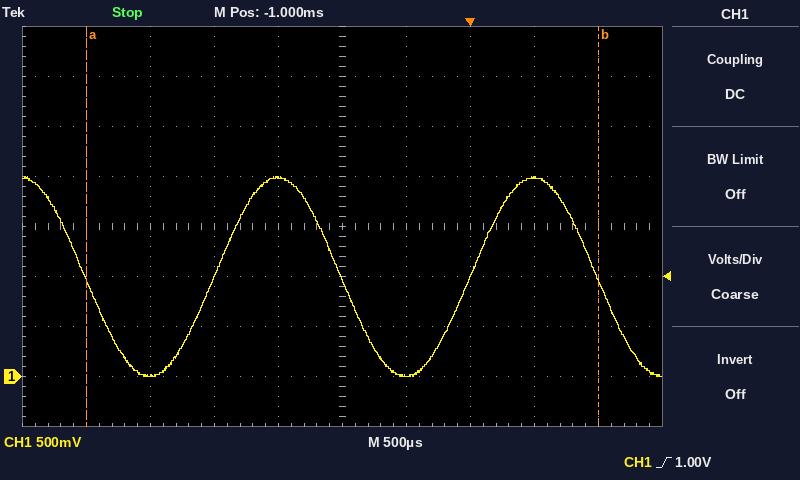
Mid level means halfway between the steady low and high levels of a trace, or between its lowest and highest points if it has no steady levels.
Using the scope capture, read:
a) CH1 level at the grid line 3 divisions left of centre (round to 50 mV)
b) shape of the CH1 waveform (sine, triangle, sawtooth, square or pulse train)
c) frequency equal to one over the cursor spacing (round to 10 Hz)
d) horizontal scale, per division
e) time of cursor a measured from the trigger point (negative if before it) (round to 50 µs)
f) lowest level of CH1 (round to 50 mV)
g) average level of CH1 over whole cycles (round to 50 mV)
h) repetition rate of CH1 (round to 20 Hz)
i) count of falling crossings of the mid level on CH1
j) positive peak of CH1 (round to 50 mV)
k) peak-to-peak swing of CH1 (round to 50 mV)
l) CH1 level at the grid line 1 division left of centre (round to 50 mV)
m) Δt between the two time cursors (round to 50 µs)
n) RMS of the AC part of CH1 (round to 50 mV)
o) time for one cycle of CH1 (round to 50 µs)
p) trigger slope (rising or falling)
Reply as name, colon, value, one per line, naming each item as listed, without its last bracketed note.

CH1 level at the grid line 3 divisions left of centre: 0 mV
shape of the CH1 waveform: sine
frequency equal to one over the cursor spacing: 250 Hz
horizontal scale, per division: 500 µs
time of cursor a measured from the trigger point (negative if before it): -3.00 ms
lowest level of CH1: 0 mV
average level of CH1 over whole cycles: 1.00 V
repetition rate of CH1: 500 Hz
count of falling crossings of the mid level on CH1: 3
positive peak of CH1: 2.00 V
peak-to-peak swing of CH1: 2.00 V
CH1 level at the grid line 1 division left of centre: 2.00 V
Δt between the two time cursors: 4.00 ms
RMS of the AC part of CH1: 700 mV
time for one cycle of CH1: 2.00 ms
trigger slope: rising
